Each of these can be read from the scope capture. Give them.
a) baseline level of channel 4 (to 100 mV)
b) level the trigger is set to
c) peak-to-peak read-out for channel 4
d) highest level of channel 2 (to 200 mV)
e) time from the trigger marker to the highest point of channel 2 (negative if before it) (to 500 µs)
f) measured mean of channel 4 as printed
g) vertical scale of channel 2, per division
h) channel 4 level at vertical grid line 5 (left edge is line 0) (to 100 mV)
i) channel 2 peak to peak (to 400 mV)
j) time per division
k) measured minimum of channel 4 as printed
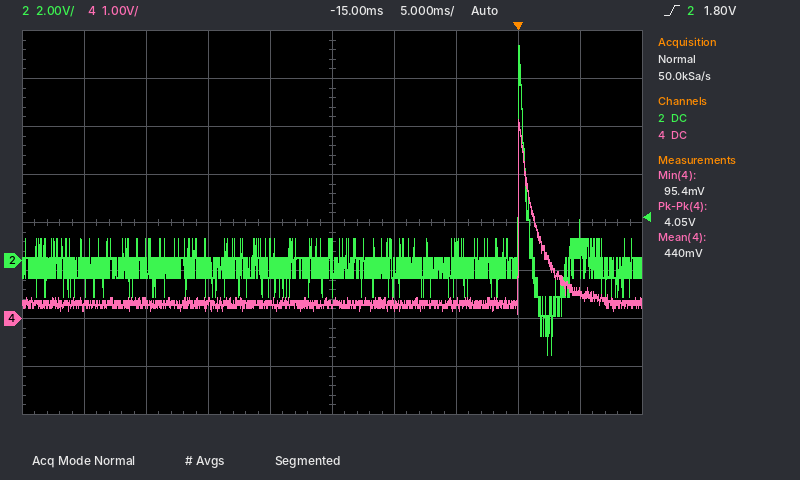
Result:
300 mV
1.80 V
4.05 V
9.0 V
0.0 ms
440 mV
2 V
300 mV
12.8 V
5 ms
95.4 mV
